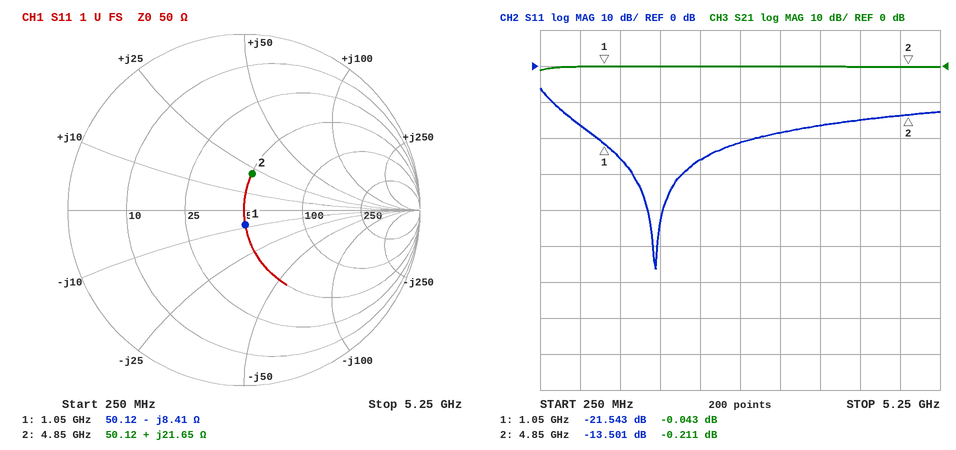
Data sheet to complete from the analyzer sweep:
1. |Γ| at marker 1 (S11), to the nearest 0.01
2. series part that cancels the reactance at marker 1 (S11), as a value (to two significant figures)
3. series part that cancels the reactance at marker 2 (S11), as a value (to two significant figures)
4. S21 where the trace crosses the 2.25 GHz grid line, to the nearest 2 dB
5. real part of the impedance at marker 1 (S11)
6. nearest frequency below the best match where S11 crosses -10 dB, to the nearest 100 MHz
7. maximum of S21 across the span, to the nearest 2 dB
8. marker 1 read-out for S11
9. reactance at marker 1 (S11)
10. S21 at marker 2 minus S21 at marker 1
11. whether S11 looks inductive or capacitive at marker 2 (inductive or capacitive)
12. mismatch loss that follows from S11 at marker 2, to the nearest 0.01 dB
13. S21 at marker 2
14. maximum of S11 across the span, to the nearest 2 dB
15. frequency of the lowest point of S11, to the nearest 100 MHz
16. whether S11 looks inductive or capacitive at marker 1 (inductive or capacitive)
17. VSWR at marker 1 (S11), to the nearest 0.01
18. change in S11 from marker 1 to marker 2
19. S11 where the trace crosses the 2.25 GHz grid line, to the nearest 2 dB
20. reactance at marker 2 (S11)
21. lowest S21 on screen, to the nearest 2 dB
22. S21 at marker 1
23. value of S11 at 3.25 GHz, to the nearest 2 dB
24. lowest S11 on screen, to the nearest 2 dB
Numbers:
0.08
1.3 nH
1.5 pF
0 dB
50.12 Ω
400 MHz
0 dB
-21.543 dB
-8.41 Ω
-0.168 dB
inductive
0.20 dB
-0.211 dB
-6 dB
1.7 GHz
capacitive
1.18
8.042 dB
-26 dB
+21.65 Ω
-2 dB
-0.043 dB
-18 dB
-56 dB
